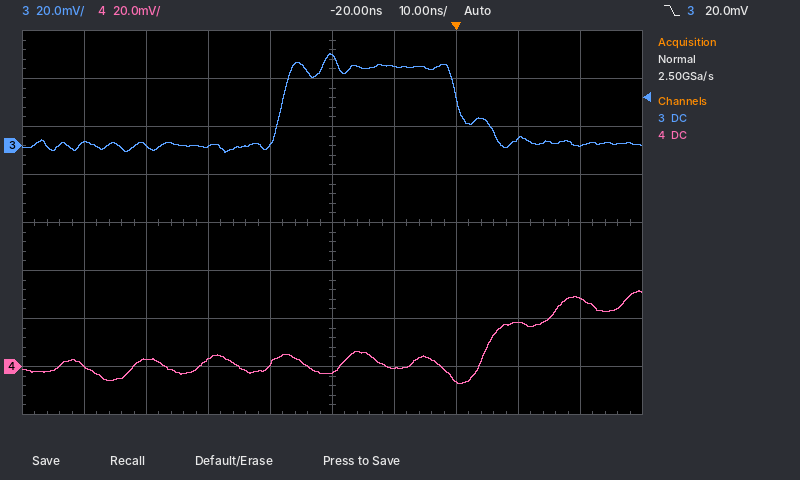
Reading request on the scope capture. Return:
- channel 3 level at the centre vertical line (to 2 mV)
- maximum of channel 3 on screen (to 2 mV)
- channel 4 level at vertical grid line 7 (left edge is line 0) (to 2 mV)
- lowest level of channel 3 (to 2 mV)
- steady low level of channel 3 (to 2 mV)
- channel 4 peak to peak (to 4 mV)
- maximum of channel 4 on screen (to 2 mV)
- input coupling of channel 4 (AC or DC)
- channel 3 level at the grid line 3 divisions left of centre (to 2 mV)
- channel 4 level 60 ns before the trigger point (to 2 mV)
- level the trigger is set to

38 mV
38 mV
-6 mV
-2 mV
0 mV
40 mV
32 mV
DC
0 mV
0 mV
20.0 mV
